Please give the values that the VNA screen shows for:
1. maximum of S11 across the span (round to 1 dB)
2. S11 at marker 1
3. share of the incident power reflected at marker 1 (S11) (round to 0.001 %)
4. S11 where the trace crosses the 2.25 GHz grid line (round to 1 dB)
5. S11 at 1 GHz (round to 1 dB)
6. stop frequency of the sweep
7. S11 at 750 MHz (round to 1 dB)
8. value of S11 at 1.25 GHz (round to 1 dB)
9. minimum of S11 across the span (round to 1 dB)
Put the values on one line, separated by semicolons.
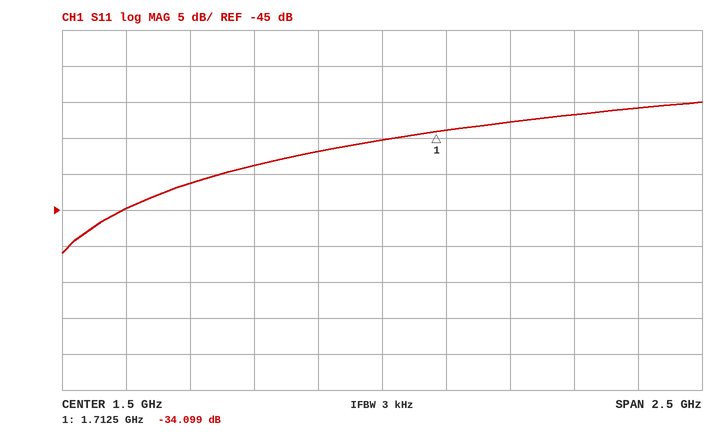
-30 dB; -34.099 dB; 0.039 %; -32 dB; -39 dB; 2.75 GHz; -41 dB; -37 dB; -51 dB
